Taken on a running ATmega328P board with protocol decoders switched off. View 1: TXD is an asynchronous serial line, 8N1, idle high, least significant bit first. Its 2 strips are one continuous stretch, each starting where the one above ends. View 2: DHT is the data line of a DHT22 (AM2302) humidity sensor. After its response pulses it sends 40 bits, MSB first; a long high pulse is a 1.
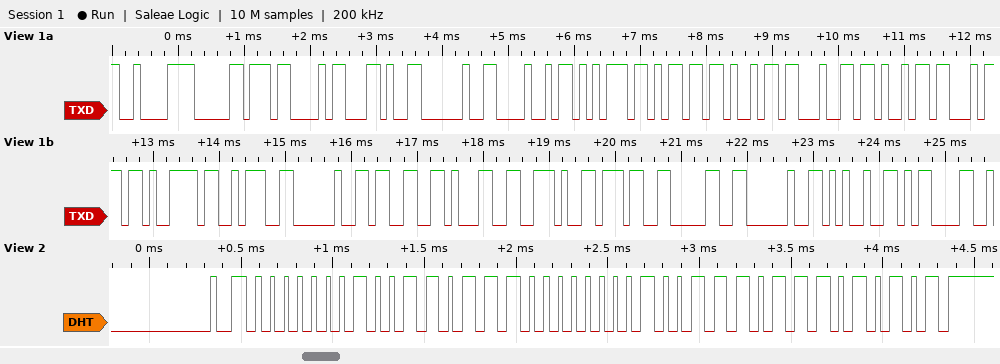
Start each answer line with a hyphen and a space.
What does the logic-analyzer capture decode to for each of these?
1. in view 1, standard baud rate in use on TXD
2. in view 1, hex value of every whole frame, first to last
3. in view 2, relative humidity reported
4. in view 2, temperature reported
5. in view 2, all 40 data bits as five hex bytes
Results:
- 9600 baud
- C2 B0 43 2C 20 48 75 6D 69 64 69 74 79 3A 20 33 31 2E 37 30 20 25 0D
- 31.1 %
- 15.7 °C
- 01 37 00 9D D5
